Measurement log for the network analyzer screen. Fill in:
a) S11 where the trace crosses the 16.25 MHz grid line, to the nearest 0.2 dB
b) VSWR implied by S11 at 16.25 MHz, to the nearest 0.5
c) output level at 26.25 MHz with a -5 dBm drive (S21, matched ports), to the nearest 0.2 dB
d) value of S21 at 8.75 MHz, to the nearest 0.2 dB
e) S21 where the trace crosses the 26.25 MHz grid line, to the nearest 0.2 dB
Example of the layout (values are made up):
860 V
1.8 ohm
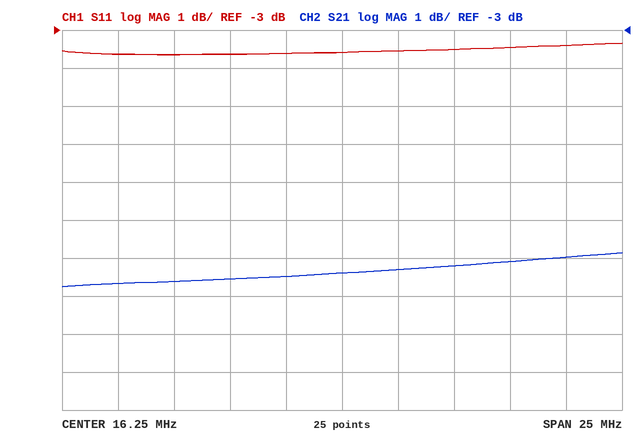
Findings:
-3.6 dB
5.0
-14.0 dBm
-9.6 dB
-9.0 dB
